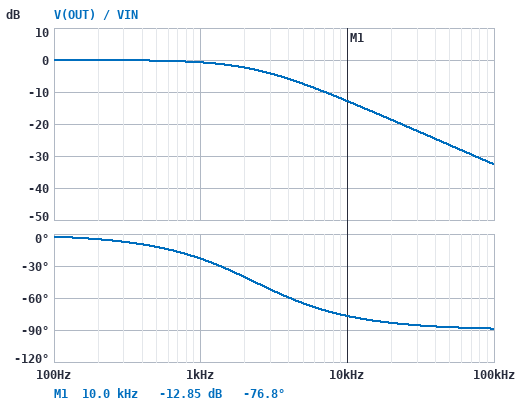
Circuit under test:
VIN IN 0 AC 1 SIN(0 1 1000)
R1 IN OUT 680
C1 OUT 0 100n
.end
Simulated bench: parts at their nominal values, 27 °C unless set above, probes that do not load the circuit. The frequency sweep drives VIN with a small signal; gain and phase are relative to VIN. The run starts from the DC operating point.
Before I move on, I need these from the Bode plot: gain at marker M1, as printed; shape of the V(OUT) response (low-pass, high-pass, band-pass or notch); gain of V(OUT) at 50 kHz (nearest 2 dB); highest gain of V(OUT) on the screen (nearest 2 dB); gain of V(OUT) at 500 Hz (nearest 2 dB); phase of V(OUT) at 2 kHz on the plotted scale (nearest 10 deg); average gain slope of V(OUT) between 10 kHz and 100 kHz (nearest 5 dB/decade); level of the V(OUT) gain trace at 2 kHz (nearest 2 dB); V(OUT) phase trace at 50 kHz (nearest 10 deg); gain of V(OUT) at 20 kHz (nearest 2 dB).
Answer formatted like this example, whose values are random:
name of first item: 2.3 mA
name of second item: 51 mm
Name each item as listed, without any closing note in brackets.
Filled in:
gain at marker M1, as printed: -12.85 dB
shape of the V(OUT) response: low-pass
gain of V(OUT) at 50 kHz: -26 dB
highest gain of V(OUT) on the screen: 0 dB
gain of V(OUT) at 500 Hz: 0 dB
phase of V(OUT) at 2 kHz on the plotted scale: -40 deg
average gain slope of V(OUT) between 10 kHz and 100 kHz: -20 dB/decade
level of the V(OUT) gain trace at 2 kHz: -2 dB
V(OUT) phase trace at 50 kHz: -90 deg
gain of V(OUT) at 20 kHz: -18 dB
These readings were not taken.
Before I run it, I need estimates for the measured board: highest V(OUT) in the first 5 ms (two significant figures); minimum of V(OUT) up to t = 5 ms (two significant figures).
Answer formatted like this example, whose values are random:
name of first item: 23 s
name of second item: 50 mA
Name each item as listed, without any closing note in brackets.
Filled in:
highest V(OUT) in the first 5 ms: 920 mV
minimum of V(OUT) up to t = 5 ms: -920 mV
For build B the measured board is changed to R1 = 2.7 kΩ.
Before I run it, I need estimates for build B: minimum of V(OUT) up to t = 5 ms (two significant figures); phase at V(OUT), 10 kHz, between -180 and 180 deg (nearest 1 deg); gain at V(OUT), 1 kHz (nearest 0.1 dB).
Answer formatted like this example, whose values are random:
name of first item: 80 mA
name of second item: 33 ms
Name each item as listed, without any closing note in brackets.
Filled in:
minimum of V(OUT) up to t = 5 ms: -510 mV
phase at V(OUT), 10 kHz, between -180 and 180 deg: -87 deg
gain at V(OUT), 1 kHz: -5.9 dB
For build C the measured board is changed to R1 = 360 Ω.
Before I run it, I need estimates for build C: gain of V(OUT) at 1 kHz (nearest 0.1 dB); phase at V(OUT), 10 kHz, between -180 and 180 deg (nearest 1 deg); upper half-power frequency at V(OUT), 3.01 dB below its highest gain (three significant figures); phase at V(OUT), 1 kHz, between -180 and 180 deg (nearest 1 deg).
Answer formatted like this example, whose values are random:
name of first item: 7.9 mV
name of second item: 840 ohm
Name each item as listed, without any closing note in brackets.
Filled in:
gain of V(OUT) at 1 kHz: -0.2 dB
phase at V(OUT), 10 kHz, between -180 and 180 deg: -66 deg
upper half-power frequency at V(OUT), 3.01 dB below its highest gain: 4.42 kHz
phase at V(OUT), 1 kHz, between -180 and 180 deg: -13 deg
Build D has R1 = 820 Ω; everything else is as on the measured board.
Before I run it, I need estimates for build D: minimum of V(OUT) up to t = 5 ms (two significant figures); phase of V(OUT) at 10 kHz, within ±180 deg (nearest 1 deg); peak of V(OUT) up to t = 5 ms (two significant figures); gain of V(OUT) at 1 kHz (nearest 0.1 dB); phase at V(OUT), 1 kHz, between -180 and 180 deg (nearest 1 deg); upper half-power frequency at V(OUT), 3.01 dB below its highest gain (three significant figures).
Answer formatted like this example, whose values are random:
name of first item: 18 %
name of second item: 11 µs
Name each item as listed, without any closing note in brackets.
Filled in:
minimum of V(OUT) up to t = 5 ms: -890 mV
phase of V(OUT) at 10 kHz, within ±180 deg: -79 deg
peak of V(OUT) up to t = 5 ms: 900 mV
gain of V(OUT) at 1 kHz: -1.0 dB
phase at V(OUT), 1 kHz, between -180 and 180 deg: -27 deg
upper half-power frequency at V(OUT), 3.01 dB below its highest gain: 1.94 kHz
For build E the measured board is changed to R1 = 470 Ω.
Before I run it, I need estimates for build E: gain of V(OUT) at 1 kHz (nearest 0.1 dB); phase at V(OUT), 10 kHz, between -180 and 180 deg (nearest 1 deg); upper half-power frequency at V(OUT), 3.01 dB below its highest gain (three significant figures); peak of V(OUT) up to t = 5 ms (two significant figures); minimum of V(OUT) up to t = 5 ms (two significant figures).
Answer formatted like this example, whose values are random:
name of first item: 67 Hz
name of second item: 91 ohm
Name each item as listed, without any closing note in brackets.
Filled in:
gain of V(OUT) at 1 kHz: -0.4 dB
phase at V(OUT), 10 kHz, between -180 and 180 deg: -71 deg
upper half-power frequency at V(OUT), 3.01 dB below its highest gain: 3.39 kHz
peak of V(OUT) up to t = 5 ms: 960 mV
minimum of V(OUT) up to t = 5 ms: -960 mV
